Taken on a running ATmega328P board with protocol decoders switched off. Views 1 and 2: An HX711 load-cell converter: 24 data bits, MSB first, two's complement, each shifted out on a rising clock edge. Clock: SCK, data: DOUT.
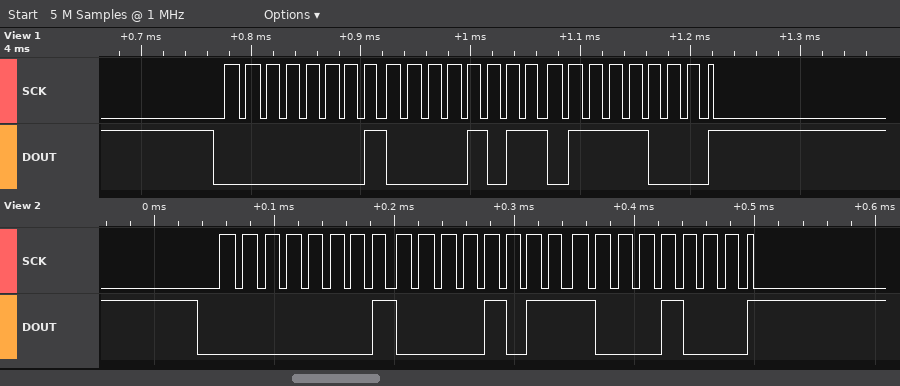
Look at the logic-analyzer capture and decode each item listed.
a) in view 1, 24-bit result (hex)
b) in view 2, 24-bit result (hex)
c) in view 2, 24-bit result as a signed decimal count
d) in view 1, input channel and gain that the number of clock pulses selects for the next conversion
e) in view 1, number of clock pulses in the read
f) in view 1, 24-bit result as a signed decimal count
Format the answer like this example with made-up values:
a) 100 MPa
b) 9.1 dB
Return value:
a) 0x010B78
b) 0x010B88
c) 68488
d) channel A, gain 128
e) 25
f) 68472
